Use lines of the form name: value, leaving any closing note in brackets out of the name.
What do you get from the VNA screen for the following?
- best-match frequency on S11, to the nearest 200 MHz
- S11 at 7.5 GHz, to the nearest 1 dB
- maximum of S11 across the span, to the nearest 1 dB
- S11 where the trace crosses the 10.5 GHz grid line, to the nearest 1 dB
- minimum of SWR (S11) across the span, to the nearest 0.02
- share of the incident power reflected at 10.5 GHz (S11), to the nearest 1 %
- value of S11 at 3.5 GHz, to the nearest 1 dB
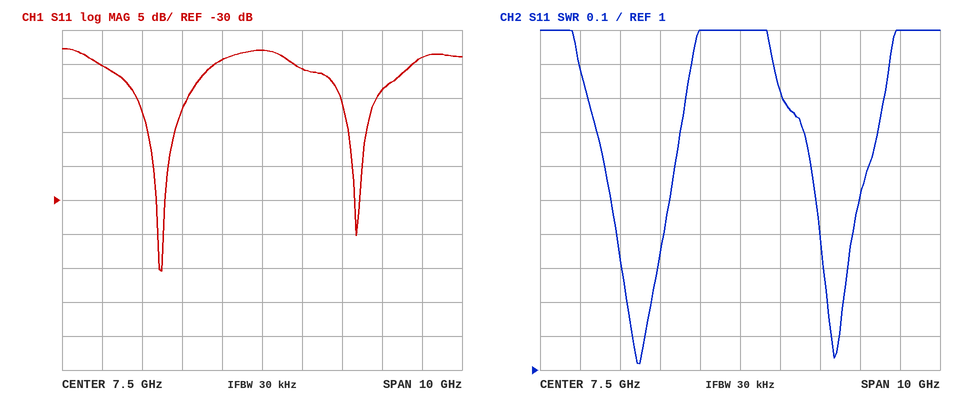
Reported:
best-match frequency on S11, to the nearest 200 MHz: 5.0 GHz
S11 at 7.5 GHz, to the nearest 1 dB: -8 dB
maximum of S11 across the span, to the nearest 1 dB: -8 dB
S11 where the trace crosses the 10.5 GHz grid line, to the nearest 1 dB: -14 dB
minimum of SWR (S11) across the span, to the nearest 0.02: 1.02
share of the incident power reflected at 10.5 GHz (S11), to the nearest 1 %: 4 %
value of S11 at 3.5 GHz, to the nearest 1 dB: -10 dB
